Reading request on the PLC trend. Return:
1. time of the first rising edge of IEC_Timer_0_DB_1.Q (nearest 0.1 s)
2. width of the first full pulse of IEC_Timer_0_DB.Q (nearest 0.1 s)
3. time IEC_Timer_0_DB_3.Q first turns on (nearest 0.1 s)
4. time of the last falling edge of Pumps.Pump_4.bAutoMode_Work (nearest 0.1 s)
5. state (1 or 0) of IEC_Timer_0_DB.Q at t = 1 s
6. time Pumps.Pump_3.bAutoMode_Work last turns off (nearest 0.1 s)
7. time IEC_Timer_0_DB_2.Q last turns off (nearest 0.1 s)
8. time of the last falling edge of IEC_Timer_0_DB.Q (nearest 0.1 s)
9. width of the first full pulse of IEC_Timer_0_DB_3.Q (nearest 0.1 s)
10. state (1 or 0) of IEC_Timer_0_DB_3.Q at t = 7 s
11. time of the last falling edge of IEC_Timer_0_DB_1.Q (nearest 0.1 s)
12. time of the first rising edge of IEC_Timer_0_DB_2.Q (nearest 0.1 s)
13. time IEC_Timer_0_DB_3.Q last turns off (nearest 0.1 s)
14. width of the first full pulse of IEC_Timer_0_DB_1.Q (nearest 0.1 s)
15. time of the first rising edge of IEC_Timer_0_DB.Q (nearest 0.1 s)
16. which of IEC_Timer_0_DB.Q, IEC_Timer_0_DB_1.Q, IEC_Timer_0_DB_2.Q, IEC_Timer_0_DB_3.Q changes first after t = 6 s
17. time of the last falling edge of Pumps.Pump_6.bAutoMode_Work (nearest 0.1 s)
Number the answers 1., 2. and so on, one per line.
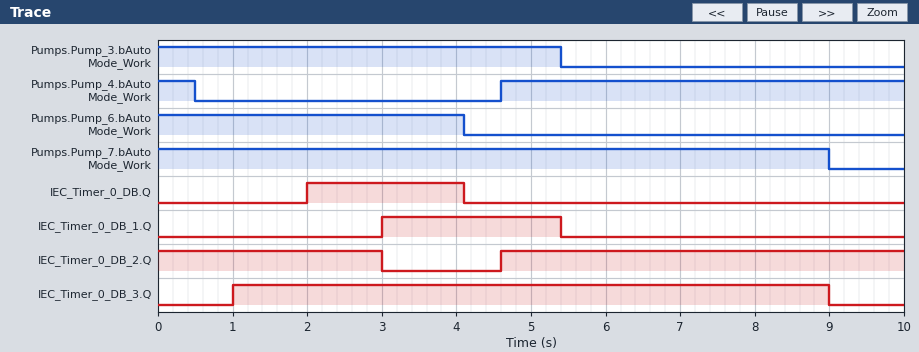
1. 3.0 s
2. 2.1 s
3. 1.0 s
4. 0.5 s
5. 0
6. 5.4 s
7. 3.0 s
8. 4.1 s
9. 8.0 s
10. 1
11. 5.4 s
12. 4.6 s
13. 9.0 s
14. 2.4 s
15. 2.0 s
16. IEC_Timer_0_DB_3.Q
17. 4.1 s
